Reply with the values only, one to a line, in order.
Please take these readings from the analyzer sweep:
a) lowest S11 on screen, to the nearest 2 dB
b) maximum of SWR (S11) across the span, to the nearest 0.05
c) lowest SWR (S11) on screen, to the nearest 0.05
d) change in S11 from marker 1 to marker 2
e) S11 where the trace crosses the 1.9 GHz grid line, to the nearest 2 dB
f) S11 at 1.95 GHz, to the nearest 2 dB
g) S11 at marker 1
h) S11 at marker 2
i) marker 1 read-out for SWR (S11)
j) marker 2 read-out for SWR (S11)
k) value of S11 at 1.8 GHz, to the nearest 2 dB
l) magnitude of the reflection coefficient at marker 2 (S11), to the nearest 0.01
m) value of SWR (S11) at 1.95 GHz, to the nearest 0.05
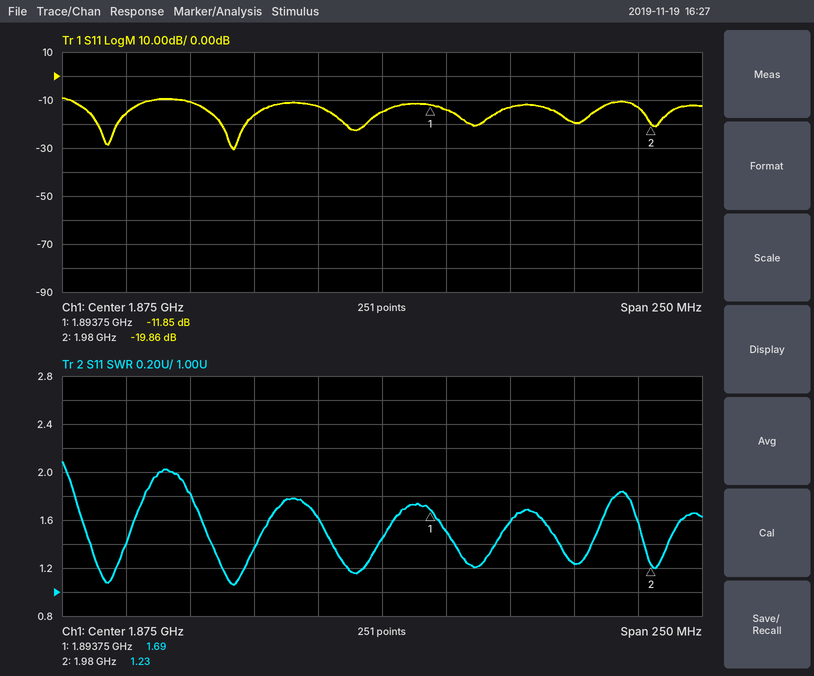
-30 dB
2.10
1.05
-8.01 dB
-14 dB
-20 dB
-11.85 dB
-19.86 dB
1.69
1.23
-10 dB
0.10
1.25
